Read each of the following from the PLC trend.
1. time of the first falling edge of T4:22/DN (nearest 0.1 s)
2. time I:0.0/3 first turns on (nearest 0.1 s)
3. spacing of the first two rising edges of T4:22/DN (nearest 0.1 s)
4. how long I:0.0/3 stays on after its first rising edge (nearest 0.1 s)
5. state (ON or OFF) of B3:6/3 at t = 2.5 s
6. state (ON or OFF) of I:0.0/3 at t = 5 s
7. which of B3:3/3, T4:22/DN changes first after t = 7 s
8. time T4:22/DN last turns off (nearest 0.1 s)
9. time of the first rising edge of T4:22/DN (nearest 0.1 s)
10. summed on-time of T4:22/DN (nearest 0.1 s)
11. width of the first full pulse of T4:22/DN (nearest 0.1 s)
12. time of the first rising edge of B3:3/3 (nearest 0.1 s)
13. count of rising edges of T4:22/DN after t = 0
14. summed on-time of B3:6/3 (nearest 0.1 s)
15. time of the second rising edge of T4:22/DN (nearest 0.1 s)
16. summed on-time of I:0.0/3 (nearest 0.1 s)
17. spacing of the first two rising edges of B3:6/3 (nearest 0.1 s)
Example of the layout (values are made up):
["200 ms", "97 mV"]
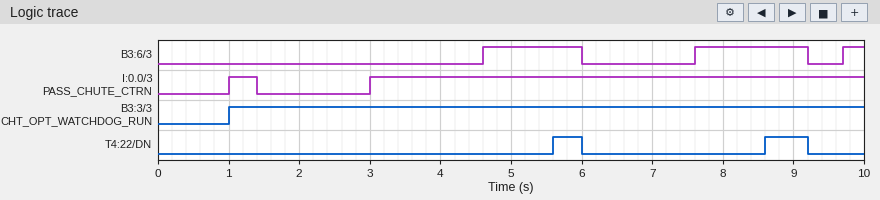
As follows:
["6.0 s", "1.0 s", "3.0 s", "0.4 s", "OFF", "ON", "T4:22/DN", "9.2 s", "5.6 s", "1.0 s", "0.4 s", "1.0 s", "2", "3.3 s", "8.6 s", "7.4 s", "3.0 s"]
